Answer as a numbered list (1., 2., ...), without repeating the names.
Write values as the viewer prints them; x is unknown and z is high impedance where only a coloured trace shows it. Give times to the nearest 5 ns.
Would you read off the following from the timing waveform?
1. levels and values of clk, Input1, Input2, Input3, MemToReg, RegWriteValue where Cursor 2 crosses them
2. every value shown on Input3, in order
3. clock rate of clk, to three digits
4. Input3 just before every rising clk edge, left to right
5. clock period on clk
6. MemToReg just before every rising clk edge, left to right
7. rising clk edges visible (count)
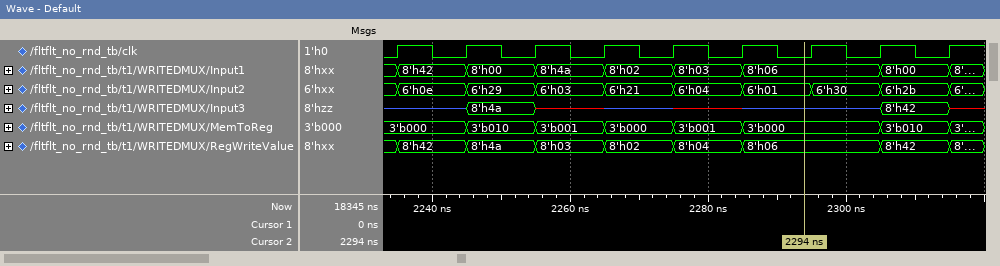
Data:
1. clk=0, Input1=8'h06, Input2=6'h01, Input3=z, MemToReg=3'b000, RegWriteValue=8'h06
2. z, 8'h4a, x, z, x, z, 8'h42, x
3. 100 MHz
4. z, z, 8'h4a, x, z, x, z, z, 8'h42
5. 10 ns
6. 3'b000, 3'b000, 3'b010, 3'b001, 3'b000, 3'b001, 3'b000, 3'b000, 3'b010
7. 9
